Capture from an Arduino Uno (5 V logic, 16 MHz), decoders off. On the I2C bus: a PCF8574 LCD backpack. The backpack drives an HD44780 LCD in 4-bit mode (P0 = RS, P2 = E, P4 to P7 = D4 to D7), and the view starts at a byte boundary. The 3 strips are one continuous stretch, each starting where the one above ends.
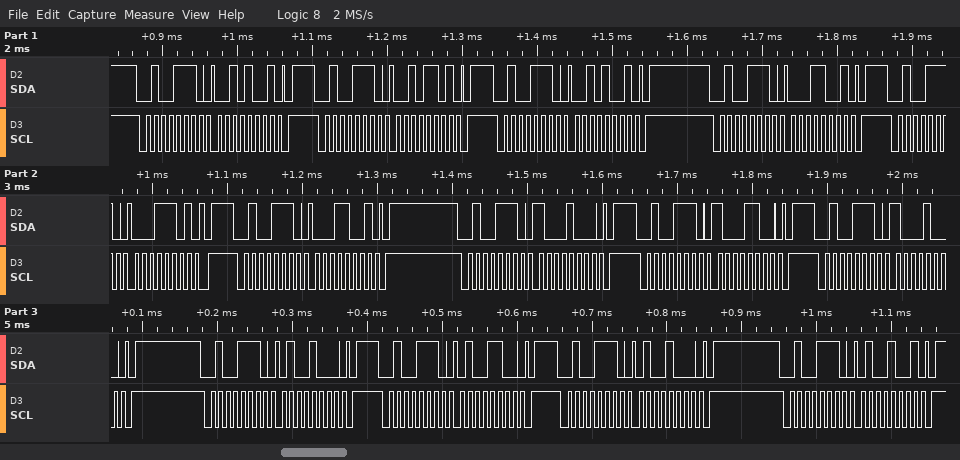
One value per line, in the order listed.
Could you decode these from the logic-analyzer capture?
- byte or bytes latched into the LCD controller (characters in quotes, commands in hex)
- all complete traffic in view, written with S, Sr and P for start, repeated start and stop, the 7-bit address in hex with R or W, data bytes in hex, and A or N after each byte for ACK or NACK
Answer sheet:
'!' 0x84
S 27W A 29 A P S 27W A 2D A P S 27W A 29 A P S 27W A 19 A P S 27W A 1D A P S 27W A 19 A P S 27W A 88 A P S 27W A 8C A P S 27W A 88 A P S 27W A 48 A P S 27W A 4C A P S 27W A 48 A P S 27W A 49 A P
